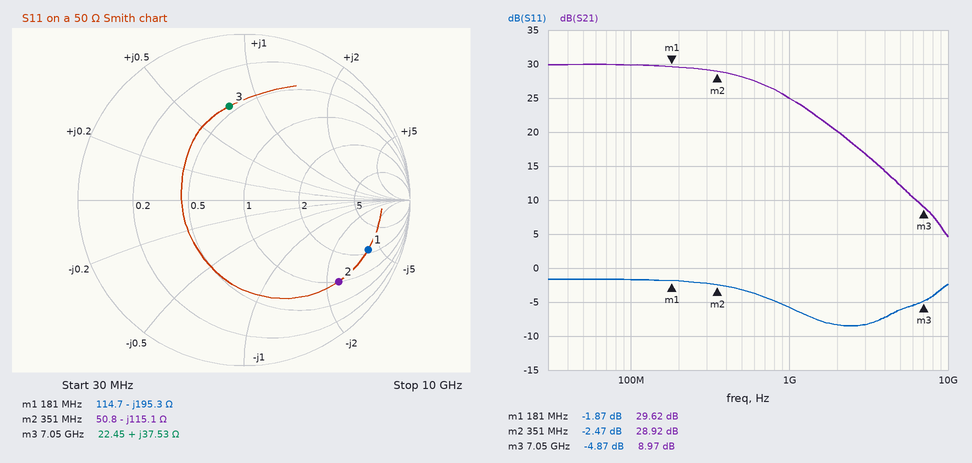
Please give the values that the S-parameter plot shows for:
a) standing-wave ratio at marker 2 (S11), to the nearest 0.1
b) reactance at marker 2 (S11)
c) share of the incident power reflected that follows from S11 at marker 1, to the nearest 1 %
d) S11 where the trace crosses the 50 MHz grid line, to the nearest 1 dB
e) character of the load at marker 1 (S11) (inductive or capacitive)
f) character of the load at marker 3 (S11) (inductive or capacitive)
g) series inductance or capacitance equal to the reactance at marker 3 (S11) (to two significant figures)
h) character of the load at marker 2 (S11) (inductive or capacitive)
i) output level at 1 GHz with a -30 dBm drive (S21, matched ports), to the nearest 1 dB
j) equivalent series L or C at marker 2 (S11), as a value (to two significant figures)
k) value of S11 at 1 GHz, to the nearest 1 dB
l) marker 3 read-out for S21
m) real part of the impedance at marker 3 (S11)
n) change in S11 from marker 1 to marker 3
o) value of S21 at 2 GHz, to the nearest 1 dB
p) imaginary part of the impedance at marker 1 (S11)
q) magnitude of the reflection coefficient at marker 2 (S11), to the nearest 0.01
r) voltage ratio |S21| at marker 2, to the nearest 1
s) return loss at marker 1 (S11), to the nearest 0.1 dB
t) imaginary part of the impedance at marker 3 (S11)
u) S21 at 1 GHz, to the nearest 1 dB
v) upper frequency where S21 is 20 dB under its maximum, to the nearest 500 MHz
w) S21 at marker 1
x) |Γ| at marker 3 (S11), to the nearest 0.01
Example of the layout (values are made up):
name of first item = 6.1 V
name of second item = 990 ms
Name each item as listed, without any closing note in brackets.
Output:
standing-wave ratio at marker 2 (S11), to the nearest 0.1 = 7.1
reactance at marker 2 = -115.1 Ω
share of the incident power reflected that follows from S11 at marker 1, to the nearest 1 % = 65 %
S11 where the trace crosses the 50 MHz grid line, to the nearest 1 dB = -2 dB
character of the load at marker 1 (S11) = capacitive
character of the load at marker 3 (S11) = inductive
series inductance or capacitance equal to the reactance at marker 3 (S11) = 850 pH
character of the load at marker 2 (S11) = capacitive
output level at 1 GHz with a -30 dBm drive (S21, matched ports), to the nearest 1 dB = -5 dBm
equivalent series L or C at marker 2 (S11), as a value = 3.9 pF
value of S11 at 1 GHz, to the nearest 1 dB = -6 dB
marker 3 read-out for S21 = 8.97 dB
real part of the impedance at marker 3 = 22.45 Ω
change in S11 from marker 1 to marker 3 = -3.00 dB
value of S21 at 2 GHz, to the nearest 1 dB = 20 dB
imaginary part of the impedance at marker 1 = -195.3 Ω
magnitude of the reflection coefficient at marker 2 (S11), to the nearest 0.01 = 0.75
voltage ratio |S21| at marker 2, to the nearest 1 = 28
return loss at marker 1 (S11), to the nearest 0.1 dB = 1.9 dB
imaginary part of the impedance at marker 3 = +37.53 Ω
S21 at 1 GHz, to the nearest 1 dB = 25 dB
upper frequency where S21 is 20 dB under its maximum, to the nearest 500 MHz = 6.5 GHz
S21 at marker 1 = 29.62 dB
|Γ| at marker 3 (S11), to the nearest 0.01 = 0.57
